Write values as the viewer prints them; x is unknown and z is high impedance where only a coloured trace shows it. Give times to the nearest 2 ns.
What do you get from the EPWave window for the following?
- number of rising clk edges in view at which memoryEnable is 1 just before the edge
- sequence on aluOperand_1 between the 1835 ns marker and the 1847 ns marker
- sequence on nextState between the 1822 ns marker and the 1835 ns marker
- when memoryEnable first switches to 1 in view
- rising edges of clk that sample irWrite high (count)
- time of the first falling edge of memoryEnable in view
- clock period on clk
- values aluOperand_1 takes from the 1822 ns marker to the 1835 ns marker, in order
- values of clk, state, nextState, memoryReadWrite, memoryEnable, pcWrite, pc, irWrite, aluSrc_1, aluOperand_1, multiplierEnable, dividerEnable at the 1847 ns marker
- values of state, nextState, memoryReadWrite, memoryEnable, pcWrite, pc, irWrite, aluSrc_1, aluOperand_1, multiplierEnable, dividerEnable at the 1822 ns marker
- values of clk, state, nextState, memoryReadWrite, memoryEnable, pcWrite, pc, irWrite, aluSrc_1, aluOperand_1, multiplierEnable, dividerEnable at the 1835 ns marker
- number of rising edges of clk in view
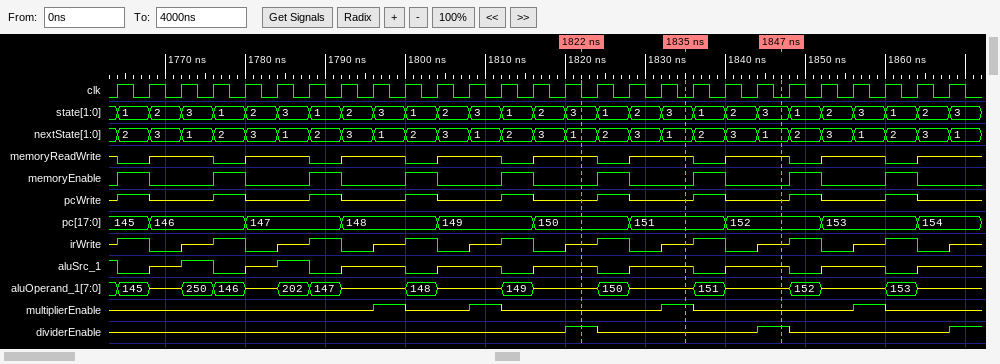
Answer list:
9
z, 151, z
1, 2, 3, 1
1764 ns
9
1768 ns
4 ns
z, 150, z
clk=0, state=3, nextState=1, memoryReadWrite=z, memoryEnable=0, pcWrite=z, pc=152, irWrite=z, aluSrc_1=z, aluOperand_1=z, multiplierEnable=z, dividerEnable=1
state=3, nextState=1, memoryReadWrite=z, memoryEnable=0, pcWrite=z, pc=150, irWrite=z, aluSrc_1=z, aluOperand_1=z, multiplierEnable=z, dividerEnable=1
clk=0, state=3, nextState=1, memoryReadWrite=z, memoryEnable=0, pcWrite=z, pc=151, irWrite=z, aluSrc_1=z, aluOperand_1=z, multiplierEnable=1, dividerEnable=z
27
